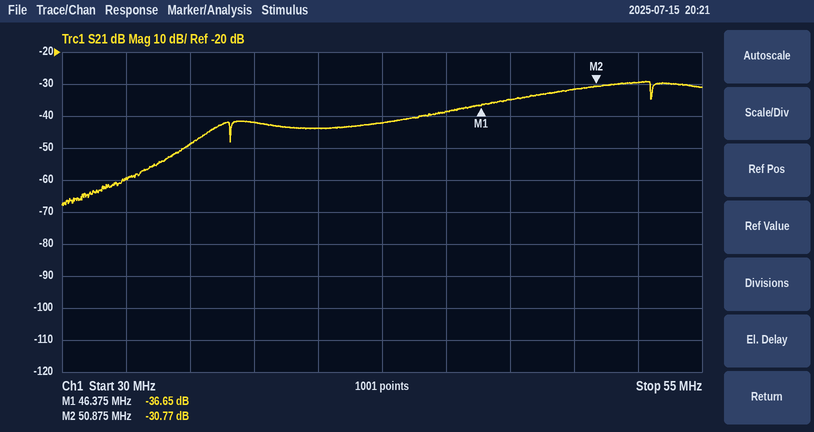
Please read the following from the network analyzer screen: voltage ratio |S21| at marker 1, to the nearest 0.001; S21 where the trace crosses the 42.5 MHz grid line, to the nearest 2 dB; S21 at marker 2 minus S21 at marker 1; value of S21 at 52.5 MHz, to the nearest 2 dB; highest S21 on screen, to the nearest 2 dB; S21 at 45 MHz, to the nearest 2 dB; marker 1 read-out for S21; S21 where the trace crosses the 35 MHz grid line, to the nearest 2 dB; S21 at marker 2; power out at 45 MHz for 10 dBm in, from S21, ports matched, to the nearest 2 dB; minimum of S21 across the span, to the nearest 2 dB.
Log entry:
0.015
-42 dB
5.88 dB
-30 dB
-30 dB
-38 dB
-36.65 dB
-48 dB
-30.77 dB
-28 dBm
-68 dB
